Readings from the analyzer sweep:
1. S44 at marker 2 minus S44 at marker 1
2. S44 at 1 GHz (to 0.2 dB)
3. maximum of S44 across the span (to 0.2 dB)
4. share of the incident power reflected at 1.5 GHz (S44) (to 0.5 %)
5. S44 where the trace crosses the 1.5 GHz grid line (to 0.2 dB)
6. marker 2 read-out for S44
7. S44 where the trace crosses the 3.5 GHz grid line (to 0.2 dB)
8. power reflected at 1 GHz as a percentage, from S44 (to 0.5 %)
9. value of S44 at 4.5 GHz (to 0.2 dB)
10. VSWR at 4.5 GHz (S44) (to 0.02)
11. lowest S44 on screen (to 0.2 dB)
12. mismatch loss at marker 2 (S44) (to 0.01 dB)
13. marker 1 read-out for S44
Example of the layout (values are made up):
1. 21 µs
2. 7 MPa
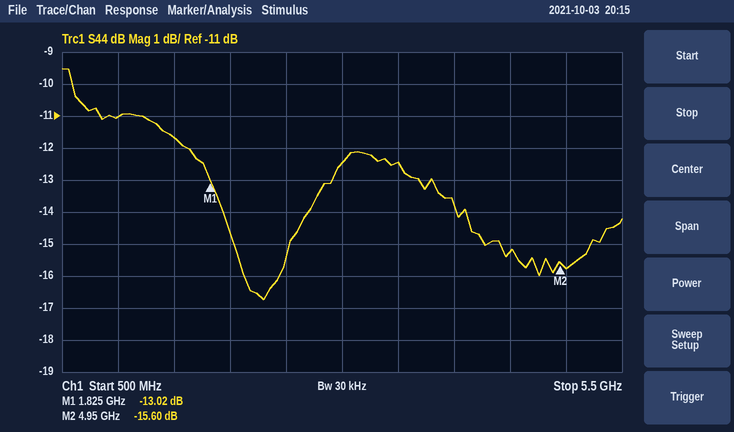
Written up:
1. -2.58 dB
2. -11.0 dB
3. -9.6 dB
4. 7.0 %
5. -11.6 dB
6. -15.60 dB
7. -12.4 dB
8. 8.0 %
9. -15.2 dB
10. 1.42
11. -16.8 dB
12. 0.12 dB
13. -13.02 dB
